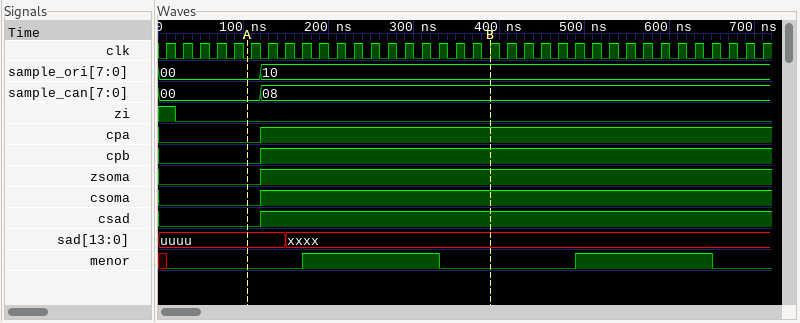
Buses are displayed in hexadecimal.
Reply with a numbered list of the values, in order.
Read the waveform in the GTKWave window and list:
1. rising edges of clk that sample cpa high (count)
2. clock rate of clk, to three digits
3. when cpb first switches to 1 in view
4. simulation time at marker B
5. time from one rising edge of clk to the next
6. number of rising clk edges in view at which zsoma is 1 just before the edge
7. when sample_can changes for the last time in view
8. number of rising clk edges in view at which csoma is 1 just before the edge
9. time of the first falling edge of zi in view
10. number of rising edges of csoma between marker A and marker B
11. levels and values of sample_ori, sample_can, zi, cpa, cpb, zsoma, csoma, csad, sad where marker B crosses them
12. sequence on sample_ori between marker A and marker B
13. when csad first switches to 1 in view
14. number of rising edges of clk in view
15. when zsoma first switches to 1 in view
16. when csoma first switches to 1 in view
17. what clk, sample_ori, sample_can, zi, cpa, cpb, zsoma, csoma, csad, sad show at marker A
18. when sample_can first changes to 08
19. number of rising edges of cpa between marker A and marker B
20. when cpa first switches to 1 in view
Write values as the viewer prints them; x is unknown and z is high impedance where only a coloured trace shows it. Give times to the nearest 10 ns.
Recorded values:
1. 30
2. 50.0 MHz
3. 120 ns
4. 390 ns
5. 20 ns
6. 30
7. 120 ns
8. 30
9. 20 ns
10. 1
11. sample_ori=10, sample_can=08, zi=0, cpa=1, cpb=1, zsoma=1, csoma=1, csad=1, sad=xxxx
12. 00, 10
13. 120 ns
14. 36
15. 120 ns
16. 120 ns
17. clk=0, sample_ori=00, sample_can=00, zi=0, cpa=0, cpb=0, zsoma=0, csoma=0, csad=0, sad=uuuu
18. 120 ns
19. 1
20. 120 ns
